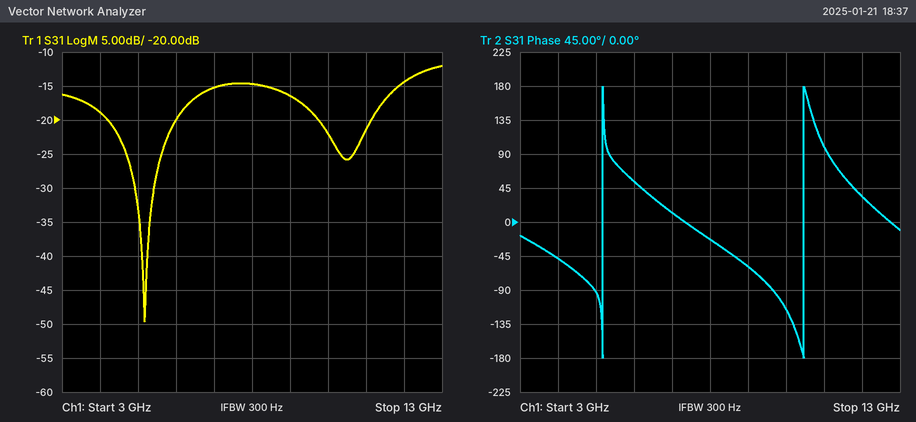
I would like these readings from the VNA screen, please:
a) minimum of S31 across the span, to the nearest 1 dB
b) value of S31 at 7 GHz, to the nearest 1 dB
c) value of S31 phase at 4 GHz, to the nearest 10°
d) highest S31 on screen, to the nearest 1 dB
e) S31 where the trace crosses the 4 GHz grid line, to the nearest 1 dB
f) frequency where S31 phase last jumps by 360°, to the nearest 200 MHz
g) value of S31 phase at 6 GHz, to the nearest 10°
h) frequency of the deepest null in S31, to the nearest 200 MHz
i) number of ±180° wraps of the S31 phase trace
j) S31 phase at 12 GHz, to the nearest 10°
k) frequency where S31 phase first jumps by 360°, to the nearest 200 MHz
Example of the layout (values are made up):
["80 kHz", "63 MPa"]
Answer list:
["-50 dB", "-15 dB", "-50°", "-12 dB", "-19 dB", "10.4 GHz", "50°", "5.2 GHz", "2", "30°", "5.2 GHz"]
